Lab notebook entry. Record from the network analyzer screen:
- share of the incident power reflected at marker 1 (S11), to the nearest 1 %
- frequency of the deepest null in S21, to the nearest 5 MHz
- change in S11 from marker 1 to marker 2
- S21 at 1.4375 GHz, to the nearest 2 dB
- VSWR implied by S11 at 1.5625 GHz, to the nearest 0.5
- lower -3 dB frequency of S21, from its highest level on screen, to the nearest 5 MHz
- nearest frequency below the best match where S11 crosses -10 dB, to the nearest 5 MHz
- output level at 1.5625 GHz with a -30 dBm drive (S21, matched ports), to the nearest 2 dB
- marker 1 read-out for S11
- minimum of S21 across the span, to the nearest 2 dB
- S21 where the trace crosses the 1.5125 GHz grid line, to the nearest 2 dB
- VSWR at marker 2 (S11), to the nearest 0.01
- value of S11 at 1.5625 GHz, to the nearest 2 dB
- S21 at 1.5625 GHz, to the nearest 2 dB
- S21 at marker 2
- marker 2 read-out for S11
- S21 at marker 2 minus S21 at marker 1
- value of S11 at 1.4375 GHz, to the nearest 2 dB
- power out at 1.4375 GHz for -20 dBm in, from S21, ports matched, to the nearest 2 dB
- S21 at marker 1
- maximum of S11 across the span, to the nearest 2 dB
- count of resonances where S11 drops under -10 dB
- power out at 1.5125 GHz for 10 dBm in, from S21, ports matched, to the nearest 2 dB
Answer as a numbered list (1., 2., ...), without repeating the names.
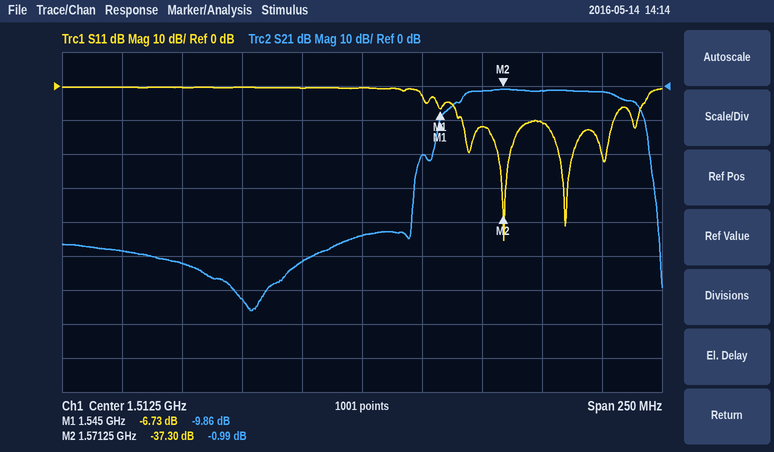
1. 21 %
2. 1.465 GHz
3. -30.57 dB
4. -52 dB
5. 1.5
6. 1.555 GHz
7. 1.555 GHz
8. -32 dBm
9. -6.73 dB
10. -66 dB
11. -44 dB
12. 1.03
13. -12 dB
14. -2 dB
15. -0.99 dB
16. -37.30 dB
17. 8.87 dB
18. 0 dB
19. -72 dBm
20. -9.86 dB
21. 0 dB
22. 5
23. -34 dBm
